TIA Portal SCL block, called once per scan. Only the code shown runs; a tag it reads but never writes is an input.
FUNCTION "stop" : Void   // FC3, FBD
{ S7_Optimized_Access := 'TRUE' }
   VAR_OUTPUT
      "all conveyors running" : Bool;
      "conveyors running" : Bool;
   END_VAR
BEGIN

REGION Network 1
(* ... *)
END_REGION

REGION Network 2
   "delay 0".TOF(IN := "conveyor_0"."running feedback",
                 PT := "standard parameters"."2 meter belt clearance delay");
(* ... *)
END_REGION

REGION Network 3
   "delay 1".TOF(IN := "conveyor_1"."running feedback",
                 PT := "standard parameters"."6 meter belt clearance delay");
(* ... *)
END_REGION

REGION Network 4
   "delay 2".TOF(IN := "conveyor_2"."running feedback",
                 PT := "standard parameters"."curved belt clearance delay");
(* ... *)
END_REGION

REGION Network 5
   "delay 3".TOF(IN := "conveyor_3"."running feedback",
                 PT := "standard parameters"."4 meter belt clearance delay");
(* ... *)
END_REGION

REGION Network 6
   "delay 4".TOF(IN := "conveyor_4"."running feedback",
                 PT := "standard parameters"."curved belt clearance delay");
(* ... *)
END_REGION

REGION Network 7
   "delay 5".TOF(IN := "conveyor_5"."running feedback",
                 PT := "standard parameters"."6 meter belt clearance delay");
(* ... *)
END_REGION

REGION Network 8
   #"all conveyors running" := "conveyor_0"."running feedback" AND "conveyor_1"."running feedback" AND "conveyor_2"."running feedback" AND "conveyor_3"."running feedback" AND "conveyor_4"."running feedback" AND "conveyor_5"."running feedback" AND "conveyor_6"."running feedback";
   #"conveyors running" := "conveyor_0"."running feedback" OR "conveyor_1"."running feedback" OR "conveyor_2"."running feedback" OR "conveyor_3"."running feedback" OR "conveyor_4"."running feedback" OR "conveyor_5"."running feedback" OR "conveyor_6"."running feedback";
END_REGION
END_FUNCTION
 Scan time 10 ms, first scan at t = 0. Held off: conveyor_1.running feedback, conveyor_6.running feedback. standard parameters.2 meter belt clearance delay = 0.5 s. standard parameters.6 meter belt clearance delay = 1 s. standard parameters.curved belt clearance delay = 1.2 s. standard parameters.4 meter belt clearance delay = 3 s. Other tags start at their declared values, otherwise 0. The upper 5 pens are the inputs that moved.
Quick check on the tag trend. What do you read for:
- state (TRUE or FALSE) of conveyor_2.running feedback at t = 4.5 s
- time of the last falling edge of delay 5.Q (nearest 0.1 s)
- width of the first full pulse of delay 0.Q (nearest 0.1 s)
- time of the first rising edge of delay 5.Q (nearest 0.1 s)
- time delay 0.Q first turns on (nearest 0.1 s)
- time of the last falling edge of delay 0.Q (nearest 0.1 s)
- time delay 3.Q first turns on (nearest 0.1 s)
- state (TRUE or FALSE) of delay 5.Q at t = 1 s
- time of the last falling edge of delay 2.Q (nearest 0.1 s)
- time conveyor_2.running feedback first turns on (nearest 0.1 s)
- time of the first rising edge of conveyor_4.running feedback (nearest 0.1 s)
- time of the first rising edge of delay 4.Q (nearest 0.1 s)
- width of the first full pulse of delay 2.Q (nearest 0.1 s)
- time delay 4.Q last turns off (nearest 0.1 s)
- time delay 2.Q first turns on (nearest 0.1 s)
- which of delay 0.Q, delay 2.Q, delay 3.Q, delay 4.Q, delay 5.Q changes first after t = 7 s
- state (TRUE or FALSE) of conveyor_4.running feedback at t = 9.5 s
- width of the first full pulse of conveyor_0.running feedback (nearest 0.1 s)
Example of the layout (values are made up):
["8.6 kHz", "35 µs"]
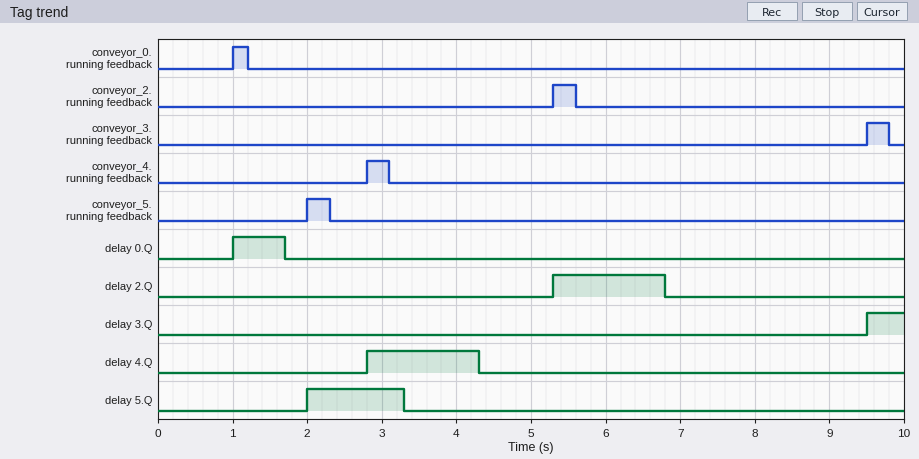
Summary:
["FALSE", "3.3 s", "0.7 s", "2.0 s", "1.0 s", "1.7 s", "9.5 s", "FALSE", "6.8 s", "5.3 s", "2.8 s", "2.8 s", "1.5 s", "4.3 s", "5.3 s", "delay 3.Q", "FALSE", "0.2 s"]
